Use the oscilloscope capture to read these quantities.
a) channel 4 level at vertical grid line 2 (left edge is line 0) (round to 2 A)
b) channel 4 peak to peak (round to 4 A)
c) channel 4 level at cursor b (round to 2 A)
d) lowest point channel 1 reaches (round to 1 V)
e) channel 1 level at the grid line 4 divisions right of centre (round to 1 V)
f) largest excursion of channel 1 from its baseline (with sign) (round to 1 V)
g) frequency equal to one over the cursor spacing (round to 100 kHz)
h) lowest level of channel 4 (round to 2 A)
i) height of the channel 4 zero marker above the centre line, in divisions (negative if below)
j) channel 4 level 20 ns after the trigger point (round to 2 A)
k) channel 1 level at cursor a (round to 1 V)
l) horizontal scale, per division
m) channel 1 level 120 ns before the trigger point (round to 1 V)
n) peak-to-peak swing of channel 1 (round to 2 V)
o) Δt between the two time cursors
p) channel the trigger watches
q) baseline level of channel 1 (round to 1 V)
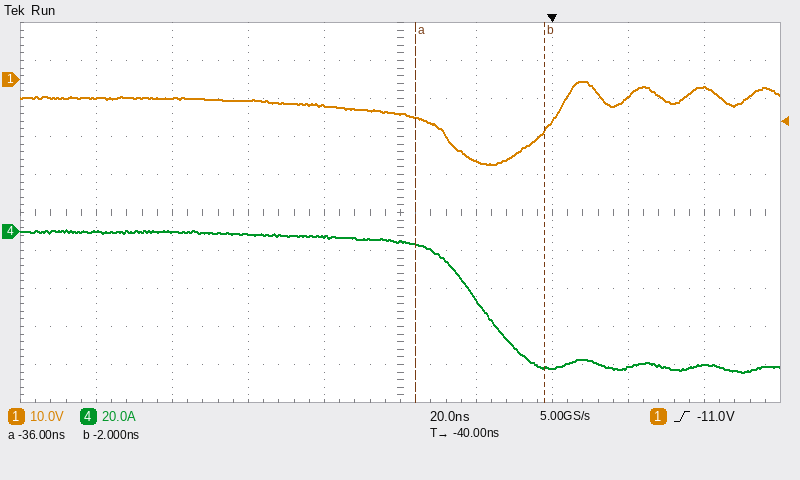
0 A
76 A
-72 A
-22 V
-2 V
-17 V
29.4 MHz
-74 A
-0.5 div
-72 A
-10 V
20 ns
-5 V
22 V
34 ns
channel 1
-5 V
